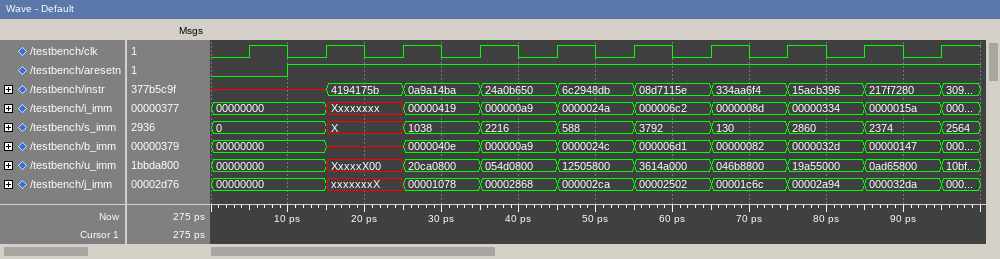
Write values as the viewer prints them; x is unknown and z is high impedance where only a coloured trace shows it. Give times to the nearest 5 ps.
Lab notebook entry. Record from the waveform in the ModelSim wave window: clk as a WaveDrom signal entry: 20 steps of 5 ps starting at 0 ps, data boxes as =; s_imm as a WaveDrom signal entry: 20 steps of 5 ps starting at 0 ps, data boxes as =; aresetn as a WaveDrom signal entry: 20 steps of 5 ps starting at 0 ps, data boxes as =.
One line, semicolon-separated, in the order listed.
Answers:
{name: 'clk', wave: '01010101010101010101'}; {name: 's_imm', wave: '=..=.=.=.=.=.=.=.=.=', data: '0 X 1038 2216 588 3792 130 2860 2374 2564'}; {name: 'aresetn', wave: '0.1.................'}
